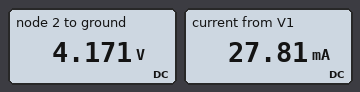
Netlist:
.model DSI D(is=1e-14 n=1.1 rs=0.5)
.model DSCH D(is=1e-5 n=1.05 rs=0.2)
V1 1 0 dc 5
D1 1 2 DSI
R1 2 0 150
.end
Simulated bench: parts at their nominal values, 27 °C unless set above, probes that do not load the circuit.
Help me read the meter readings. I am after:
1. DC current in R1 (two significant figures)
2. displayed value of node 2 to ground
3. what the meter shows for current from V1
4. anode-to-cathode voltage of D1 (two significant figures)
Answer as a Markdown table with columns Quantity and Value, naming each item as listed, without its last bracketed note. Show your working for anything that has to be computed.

| Quantity | Value |
|---|---|
| DC current in R1 | (4.171 V) / 150 Ω = 28 mA |
| displayed value of node 2 to ground | 4.171 V |
| what the meter shows for current from V1 | 27.81 mA |
| anode-to-cathode voltage of D1 | 5 V - 4.171 V = 830 mV |
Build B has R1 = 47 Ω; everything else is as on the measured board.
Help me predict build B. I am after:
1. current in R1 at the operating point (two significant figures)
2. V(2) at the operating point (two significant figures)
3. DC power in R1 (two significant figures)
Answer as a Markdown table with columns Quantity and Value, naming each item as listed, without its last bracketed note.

| Quantity | Value |
|---|---|
| current in R1 at the operating point | 87 mA |
| V(2) at the operating point | 4.1 V |
| DC power in R1 | 360 mW |
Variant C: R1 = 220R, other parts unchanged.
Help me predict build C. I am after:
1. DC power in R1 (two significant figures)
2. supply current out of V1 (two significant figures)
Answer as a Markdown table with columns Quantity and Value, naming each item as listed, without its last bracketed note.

| Quantity | Value |
|---|---|
| DC power in R1 | 80 mW |
| supply current out of V1 | 19 mA |
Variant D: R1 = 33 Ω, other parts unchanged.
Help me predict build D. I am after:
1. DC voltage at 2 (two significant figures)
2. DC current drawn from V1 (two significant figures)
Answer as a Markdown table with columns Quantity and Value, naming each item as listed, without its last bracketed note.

| Quantity | Value |
|---|---|
| DC voltage at 2 | 4.1 V |
| DC current drawn from V1 | 120 mA |
